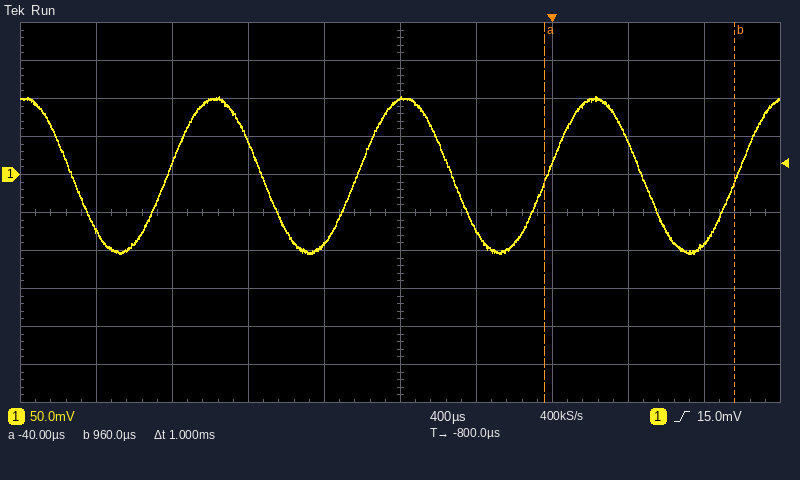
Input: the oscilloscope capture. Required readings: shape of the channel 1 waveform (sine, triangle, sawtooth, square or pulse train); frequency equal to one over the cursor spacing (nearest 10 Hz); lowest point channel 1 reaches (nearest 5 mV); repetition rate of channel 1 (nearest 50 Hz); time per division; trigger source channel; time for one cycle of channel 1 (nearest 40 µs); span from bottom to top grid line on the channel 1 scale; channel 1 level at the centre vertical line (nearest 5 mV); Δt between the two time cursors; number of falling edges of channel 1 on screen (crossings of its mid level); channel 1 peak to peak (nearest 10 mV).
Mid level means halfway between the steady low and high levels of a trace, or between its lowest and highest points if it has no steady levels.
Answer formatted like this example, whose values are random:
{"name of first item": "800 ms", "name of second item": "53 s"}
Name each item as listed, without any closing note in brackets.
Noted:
{"shape of the channel 1 waveform": "sine", "frequency equal to one over the cursor spacing": "1.00 kHz", "lowest point channel 1 reaches": "-105 mV", "repetition rate of channel 1": "1.00 kHz", "time per division": "400 µs", "trigger source channel": "channel 1", "time for one cycle of channel 1": "1.00 ms", "span from bottom to top grid line on the channel 1 scale": "500 mV", "channel 1 level at the centre vertical line": "100 mV", "Δt between the two time cursors": "1 ms", "number of falling edges of channel 1 on screen": "4", "channel 1 peak to peak": "210 mV"}
